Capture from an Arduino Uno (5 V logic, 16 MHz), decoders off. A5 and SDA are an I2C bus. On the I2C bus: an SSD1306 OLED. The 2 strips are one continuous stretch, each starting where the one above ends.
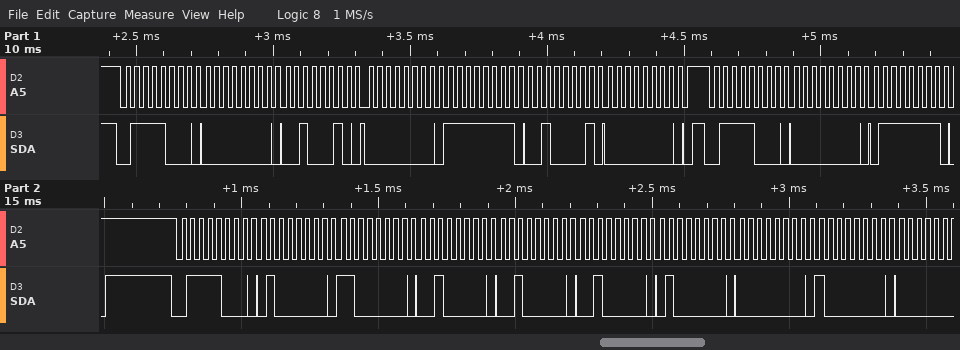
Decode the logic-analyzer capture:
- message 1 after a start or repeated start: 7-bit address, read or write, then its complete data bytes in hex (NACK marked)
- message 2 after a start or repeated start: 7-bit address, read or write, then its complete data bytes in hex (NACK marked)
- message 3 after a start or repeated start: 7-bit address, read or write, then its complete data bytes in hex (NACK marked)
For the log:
0x3C write: 00 22 00 FF 21 00
0x3C write: 00 7F
0x3C write: 40 C0 20 20 20 40 00 80
